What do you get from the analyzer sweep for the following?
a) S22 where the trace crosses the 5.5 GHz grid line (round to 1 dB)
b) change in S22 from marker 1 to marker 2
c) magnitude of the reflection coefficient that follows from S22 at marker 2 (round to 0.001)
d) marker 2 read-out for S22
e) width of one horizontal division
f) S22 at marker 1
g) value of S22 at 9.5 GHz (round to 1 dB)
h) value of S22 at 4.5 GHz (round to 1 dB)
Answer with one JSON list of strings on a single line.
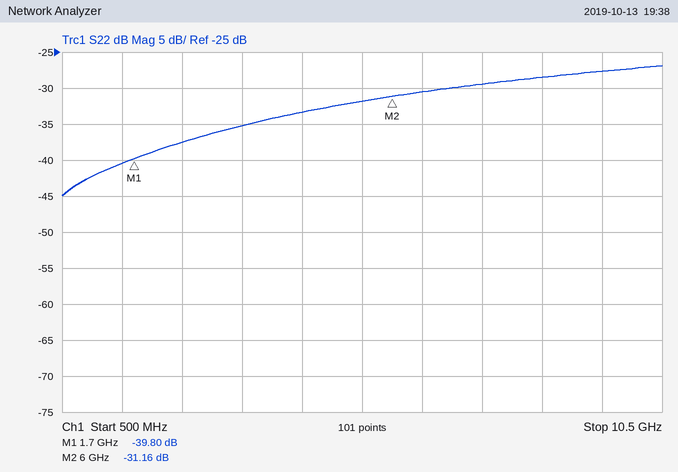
["-32 dB", "8.64 dB", "0.028", "-31.16 dB", "1 GHz", "-39.80 dB", "-28 dB", "-33 dB"]
